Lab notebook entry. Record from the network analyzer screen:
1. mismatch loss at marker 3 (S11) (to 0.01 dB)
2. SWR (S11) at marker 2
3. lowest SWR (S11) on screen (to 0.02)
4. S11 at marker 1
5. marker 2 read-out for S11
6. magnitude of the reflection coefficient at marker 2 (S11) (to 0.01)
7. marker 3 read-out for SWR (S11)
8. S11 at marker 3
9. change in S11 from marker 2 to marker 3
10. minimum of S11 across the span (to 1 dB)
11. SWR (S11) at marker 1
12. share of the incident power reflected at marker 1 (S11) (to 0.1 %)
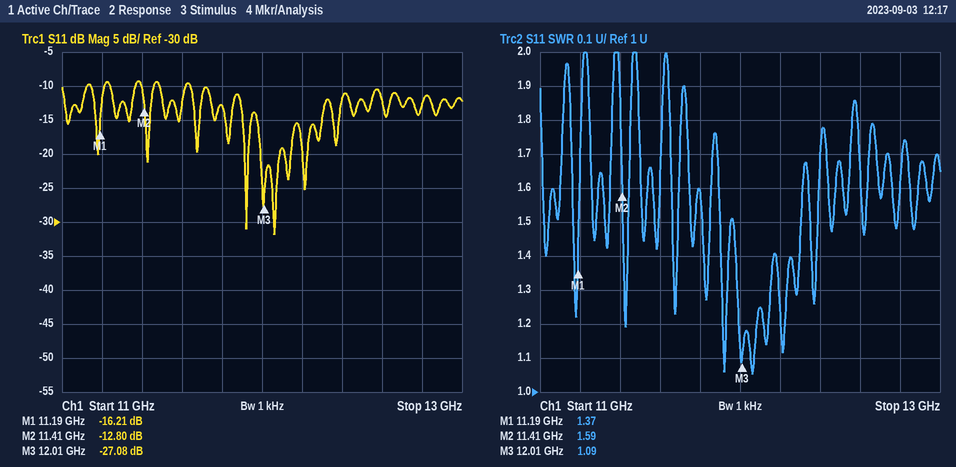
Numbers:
0.01 dB
1.59
1.06
-16.21 dB
-12.80 dB
0.23
1.09
-27.08 dB
-14.28 dB
-32 dB
1.37
2.4 %
